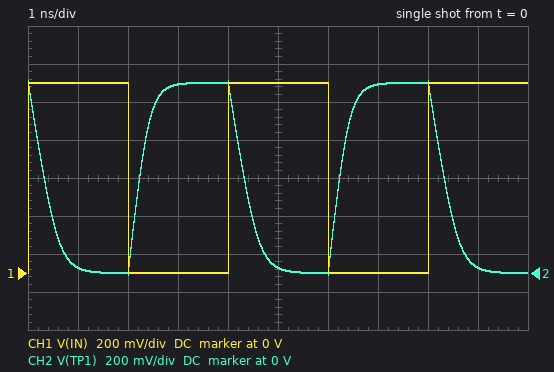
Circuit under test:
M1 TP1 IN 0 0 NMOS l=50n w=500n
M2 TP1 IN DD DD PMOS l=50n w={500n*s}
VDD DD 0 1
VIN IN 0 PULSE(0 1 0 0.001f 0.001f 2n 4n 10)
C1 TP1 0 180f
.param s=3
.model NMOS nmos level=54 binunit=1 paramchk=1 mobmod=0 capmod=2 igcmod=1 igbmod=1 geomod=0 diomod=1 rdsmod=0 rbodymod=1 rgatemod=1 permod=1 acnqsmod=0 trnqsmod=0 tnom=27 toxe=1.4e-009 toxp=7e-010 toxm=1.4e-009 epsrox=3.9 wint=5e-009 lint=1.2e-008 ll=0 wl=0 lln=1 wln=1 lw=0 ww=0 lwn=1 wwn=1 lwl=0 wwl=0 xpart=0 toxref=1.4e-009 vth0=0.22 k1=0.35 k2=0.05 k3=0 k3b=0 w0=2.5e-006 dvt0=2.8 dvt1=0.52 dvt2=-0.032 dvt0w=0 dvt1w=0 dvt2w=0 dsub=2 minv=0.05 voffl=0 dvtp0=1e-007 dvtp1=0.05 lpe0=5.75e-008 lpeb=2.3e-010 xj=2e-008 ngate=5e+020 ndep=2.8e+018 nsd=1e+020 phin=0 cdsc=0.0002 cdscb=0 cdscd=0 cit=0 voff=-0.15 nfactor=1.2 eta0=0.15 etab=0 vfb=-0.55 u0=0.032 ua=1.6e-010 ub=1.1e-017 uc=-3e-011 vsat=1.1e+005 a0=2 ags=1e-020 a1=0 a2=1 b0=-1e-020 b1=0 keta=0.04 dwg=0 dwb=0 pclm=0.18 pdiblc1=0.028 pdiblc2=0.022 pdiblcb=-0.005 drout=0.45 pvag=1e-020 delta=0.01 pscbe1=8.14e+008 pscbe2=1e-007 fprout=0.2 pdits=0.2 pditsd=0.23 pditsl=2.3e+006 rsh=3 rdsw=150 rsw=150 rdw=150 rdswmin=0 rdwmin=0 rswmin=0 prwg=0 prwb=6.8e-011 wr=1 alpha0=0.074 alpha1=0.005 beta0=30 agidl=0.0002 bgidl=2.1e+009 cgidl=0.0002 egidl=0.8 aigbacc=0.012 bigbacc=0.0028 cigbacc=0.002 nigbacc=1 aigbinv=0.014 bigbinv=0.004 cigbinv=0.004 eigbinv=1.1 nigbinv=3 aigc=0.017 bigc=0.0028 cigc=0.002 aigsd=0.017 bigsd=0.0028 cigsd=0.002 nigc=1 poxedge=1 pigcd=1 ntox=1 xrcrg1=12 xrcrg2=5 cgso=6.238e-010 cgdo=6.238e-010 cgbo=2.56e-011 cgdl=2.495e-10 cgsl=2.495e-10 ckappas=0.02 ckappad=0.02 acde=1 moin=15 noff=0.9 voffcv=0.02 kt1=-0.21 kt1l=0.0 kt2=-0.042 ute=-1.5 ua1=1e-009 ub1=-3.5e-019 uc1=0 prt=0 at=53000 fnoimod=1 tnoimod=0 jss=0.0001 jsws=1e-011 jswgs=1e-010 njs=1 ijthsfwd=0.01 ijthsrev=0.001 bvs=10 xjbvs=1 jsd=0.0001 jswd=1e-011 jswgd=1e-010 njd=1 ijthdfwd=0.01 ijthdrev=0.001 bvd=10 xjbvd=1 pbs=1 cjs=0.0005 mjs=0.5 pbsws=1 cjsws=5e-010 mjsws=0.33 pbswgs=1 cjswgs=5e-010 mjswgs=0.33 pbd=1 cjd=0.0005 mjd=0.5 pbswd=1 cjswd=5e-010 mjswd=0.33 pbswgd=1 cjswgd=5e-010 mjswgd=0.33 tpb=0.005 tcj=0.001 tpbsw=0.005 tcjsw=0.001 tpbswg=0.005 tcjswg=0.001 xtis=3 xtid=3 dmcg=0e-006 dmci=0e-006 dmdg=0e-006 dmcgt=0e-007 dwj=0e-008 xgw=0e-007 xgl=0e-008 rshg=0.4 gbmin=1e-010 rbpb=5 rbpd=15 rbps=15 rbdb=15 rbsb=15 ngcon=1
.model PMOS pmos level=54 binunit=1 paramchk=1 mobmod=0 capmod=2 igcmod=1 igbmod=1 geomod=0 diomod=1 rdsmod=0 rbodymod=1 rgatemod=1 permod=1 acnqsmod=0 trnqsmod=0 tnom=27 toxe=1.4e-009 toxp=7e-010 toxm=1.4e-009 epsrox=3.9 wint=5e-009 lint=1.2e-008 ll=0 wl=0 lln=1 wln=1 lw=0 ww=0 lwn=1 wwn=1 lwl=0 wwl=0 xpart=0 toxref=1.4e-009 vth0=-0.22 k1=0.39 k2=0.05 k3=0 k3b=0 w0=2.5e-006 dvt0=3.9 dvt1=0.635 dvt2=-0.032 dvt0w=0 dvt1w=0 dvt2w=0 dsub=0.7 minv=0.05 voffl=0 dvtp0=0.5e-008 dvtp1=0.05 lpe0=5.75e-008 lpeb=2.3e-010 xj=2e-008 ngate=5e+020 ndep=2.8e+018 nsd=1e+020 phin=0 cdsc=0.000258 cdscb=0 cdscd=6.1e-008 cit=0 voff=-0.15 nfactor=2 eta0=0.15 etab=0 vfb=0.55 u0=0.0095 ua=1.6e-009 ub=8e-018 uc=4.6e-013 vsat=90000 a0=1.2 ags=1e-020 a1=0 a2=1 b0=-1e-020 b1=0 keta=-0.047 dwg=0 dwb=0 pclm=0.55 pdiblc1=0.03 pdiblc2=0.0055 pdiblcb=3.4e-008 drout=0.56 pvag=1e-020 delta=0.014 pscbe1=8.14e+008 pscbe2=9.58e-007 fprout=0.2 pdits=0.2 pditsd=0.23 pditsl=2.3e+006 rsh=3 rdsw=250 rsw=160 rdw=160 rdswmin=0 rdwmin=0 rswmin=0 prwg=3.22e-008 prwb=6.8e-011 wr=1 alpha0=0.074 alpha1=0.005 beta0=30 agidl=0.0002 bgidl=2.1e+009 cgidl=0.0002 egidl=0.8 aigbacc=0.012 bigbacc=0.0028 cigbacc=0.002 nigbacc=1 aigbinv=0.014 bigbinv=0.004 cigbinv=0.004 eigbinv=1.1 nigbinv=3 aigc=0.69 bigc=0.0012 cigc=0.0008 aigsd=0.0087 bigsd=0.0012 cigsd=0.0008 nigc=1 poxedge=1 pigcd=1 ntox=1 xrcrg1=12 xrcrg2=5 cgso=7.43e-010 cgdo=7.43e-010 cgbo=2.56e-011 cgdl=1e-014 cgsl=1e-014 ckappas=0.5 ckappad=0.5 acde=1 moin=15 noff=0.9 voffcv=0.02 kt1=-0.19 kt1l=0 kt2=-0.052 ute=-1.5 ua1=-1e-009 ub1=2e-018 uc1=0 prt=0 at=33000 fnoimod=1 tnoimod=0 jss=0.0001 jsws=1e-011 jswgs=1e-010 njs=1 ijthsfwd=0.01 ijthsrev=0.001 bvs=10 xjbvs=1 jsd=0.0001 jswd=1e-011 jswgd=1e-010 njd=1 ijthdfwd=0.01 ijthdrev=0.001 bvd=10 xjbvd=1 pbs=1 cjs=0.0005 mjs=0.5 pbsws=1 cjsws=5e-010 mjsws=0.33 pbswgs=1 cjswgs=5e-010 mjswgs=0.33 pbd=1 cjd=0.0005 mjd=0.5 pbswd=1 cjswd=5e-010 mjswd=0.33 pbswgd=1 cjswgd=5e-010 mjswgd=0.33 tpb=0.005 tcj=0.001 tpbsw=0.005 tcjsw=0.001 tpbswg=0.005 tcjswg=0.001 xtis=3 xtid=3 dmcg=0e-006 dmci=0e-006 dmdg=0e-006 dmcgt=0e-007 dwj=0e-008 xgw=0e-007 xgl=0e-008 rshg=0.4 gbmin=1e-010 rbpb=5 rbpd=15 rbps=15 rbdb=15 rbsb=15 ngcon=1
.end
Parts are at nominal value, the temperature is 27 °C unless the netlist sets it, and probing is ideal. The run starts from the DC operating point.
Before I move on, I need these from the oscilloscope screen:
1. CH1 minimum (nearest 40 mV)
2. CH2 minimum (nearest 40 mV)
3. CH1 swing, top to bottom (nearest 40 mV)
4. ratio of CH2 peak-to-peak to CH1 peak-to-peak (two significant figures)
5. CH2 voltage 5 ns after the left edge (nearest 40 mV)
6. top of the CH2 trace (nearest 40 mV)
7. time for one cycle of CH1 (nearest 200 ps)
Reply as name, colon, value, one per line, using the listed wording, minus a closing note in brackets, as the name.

CH1 minimum: 0 V
CH2 minimum: 0 V
CH1 swing, top to bottom: 1.00 V
ratio of CH2 peak-to-peak to CH1 peak-to-peak: 1.0
CH2 voltage 5 ns after the left edge: 40 mV
top of the CH2 trace: 1.00 V
time for one cycle of CH1: 4.0 ns
